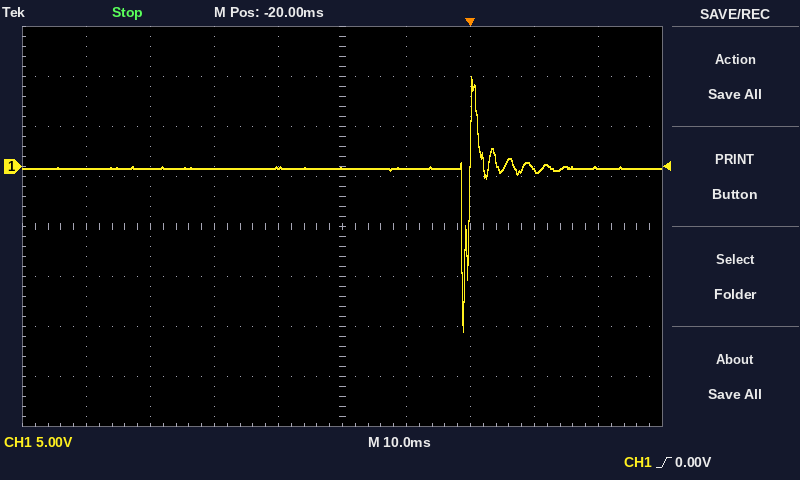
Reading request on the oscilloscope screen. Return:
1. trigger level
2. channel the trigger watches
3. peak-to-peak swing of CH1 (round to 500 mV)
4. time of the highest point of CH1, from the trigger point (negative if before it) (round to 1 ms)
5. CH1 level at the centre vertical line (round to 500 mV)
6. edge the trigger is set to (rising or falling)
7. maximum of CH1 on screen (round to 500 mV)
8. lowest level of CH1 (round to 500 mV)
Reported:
0.00 V
CH1
25.5 V
0 ms
0.0 V
rising
9.0 V
-16.5 V
